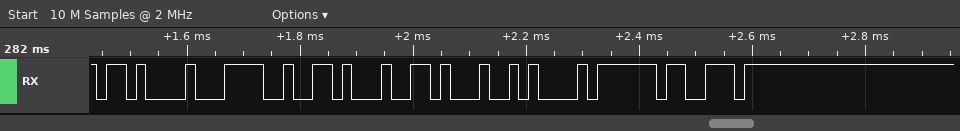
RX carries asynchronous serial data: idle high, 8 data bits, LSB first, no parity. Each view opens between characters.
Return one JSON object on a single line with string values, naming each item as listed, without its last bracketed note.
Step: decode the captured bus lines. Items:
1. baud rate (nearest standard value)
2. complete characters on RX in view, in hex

{"baud rate": "57600 baud", "complete characters on RX in view, in hex": "0B, 3C, 16, 16, 0A, BF, EE"}
